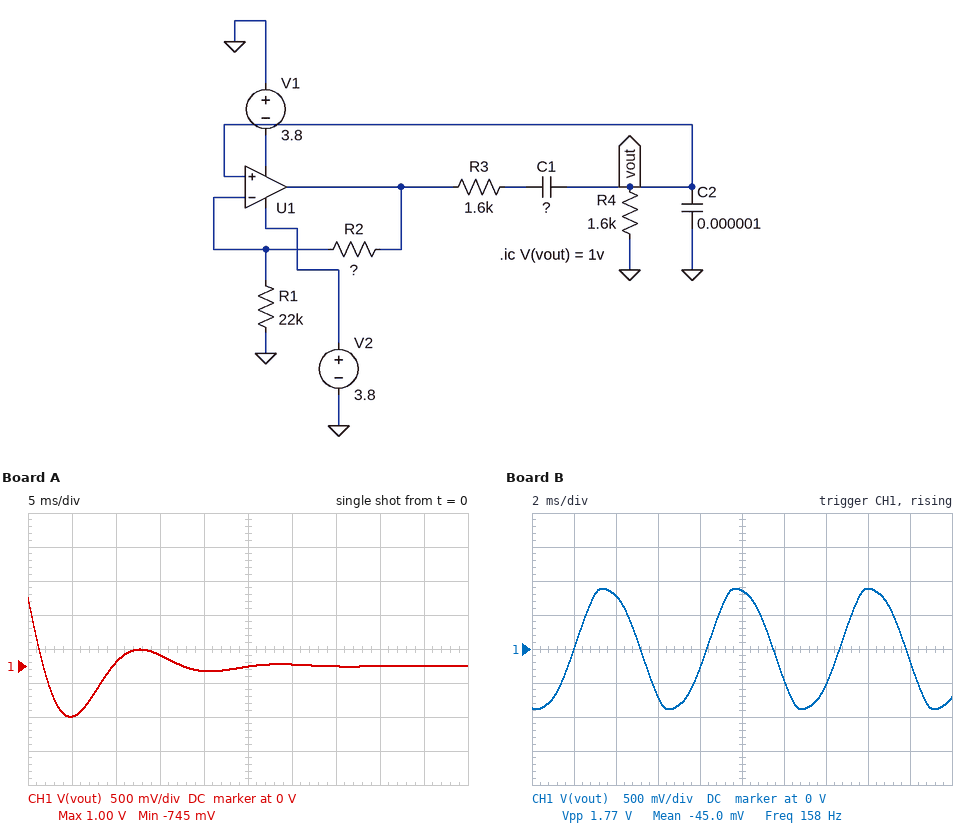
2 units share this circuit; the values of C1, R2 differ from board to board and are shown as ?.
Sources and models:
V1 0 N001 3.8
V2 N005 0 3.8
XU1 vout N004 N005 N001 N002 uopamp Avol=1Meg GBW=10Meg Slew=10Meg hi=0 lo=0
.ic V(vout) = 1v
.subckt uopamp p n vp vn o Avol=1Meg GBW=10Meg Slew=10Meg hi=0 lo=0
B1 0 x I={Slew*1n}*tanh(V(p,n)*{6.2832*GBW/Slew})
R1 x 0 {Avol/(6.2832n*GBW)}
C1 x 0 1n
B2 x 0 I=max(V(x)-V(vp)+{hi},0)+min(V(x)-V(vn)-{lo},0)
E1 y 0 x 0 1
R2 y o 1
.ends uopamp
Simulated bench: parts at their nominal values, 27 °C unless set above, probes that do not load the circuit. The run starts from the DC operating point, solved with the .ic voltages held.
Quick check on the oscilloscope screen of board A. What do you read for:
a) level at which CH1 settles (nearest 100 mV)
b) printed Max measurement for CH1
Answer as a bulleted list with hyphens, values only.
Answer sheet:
- 0 V
- 1.00 V
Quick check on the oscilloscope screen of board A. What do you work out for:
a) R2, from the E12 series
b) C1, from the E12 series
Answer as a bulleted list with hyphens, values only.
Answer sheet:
- 22 kΩ
- 2.2 µF
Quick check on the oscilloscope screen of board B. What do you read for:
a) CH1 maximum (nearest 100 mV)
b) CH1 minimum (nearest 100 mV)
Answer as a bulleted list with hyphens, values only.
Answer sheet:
- 900 mV
- -900 mV
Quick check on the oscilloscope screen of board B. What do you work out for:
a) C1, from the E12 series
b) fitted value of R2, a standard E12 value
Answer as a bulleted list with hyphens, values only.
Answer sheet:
- 390 nF
- 82 kΩ
